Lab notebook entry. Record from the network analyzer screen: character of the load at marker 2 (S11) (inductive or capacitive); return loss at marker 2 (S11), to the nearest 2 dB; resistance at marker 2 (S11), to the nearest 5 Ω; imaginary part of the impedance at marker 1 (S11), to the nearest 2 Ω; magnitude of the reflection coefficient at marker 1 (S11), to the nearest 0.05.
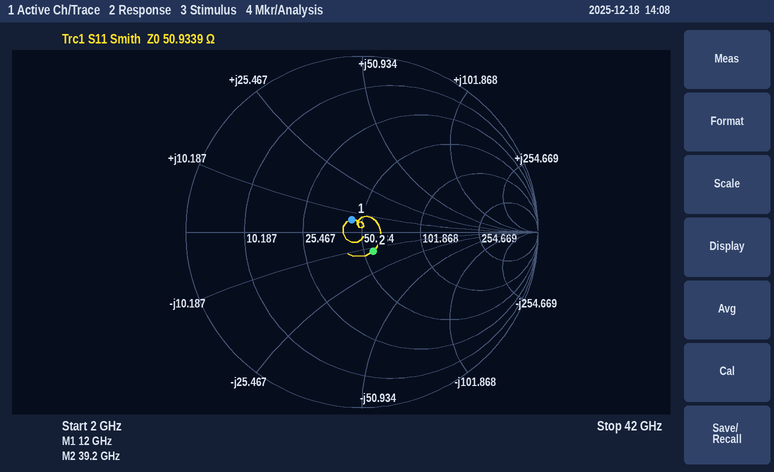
capacitive
18 dB
55 Ω
+6 Ω
0.10
